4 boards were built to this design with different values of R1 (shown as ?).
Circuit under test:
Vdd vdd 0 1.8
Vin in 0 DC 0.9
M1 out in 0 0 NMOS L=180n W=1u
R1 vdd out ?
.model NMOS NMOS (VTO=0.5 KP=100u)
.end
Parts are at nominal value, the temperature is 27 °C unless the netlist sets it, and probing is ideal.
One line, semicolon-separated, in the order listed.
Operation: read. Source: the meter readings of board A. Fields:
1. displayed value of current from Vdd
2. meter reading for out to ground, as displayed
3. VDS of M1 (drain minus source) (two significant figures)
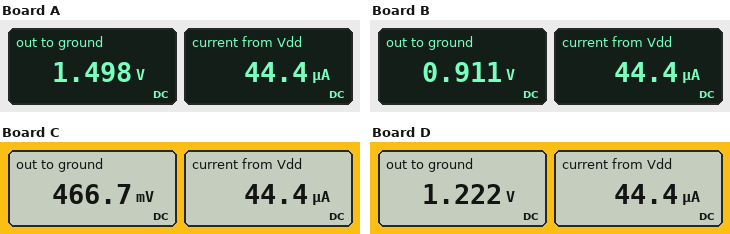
44.4 µA; 1.498 V; 1.5 V
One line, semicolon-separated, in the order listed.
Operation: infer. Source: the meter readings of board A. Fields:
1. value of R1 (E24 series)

6.8 kΩ
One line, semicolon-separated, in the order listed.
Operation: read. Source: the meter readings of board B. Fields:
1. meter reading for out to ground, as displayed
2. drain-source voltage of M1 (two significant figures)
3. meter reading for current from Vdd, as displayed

0.911 V; 910 mV; 44.4 µA
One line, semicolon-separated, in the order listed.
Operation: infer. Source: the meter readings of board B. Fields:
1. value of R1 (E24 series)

20 kΩ
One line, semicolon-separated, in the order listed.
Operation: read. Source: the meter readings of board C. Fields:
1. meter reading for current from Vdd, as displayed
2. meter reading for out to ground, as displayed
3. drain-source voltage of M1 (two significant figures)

44.4 µA; 466.7 mV; 470 mV
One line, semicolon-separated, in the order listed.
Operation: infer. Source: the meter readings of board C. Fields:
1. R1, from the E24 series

30 kΩ
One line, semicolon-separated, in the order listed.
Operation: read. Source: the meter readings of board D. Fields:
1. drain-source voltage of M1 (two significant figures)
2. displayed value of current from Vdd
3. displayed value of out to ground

1.2 V; 44.4 µA; 1.222 V
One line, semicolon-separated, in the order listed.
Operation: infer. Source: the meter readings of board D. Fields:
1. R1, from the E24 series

13 kΩ
